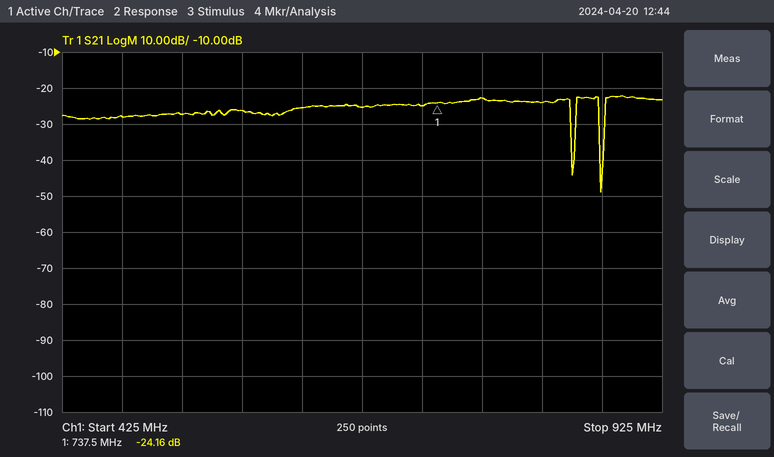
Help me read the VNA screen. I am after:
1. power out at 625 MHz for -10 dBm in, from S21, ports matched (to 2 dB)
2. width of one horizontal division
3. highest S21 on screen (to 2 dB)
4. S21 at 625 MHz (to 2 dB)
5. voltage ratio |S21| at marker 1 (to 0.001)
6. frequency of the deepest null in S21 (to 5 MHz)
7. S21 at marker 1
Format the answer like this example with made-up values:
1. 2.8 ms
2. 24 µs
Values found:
1. -36 dBm
2. 50 MHz
3. -22 dB
4. -26 dB
5. 0.062
6. 875 MHz
7. -24.16 dB
